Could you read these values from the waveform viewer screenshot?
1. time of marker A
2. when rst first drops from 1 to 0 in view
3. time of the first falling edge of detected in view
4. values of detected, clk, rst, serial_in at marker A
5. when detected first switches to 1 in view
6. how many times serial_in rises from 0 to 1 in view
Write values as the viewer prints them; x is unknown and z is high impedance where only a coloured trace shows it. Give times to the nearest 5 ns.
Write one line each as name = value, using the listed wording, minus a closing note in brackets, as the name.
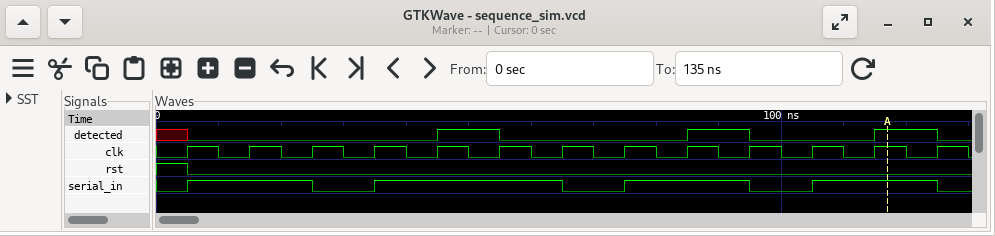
time of marker A = 115 ns
when rst first drops from 1 to 0 in view = 5 ns
time of the first falling edge of detected in view = 55 ns
values of detected, clk, rst, serial_in at marker A = detected=1, clk=1, rst=0, serial_in=1
when detected first switches to 1 in view = 45 ns
how many times serial_in rises from 0 to 1 in view = 4
